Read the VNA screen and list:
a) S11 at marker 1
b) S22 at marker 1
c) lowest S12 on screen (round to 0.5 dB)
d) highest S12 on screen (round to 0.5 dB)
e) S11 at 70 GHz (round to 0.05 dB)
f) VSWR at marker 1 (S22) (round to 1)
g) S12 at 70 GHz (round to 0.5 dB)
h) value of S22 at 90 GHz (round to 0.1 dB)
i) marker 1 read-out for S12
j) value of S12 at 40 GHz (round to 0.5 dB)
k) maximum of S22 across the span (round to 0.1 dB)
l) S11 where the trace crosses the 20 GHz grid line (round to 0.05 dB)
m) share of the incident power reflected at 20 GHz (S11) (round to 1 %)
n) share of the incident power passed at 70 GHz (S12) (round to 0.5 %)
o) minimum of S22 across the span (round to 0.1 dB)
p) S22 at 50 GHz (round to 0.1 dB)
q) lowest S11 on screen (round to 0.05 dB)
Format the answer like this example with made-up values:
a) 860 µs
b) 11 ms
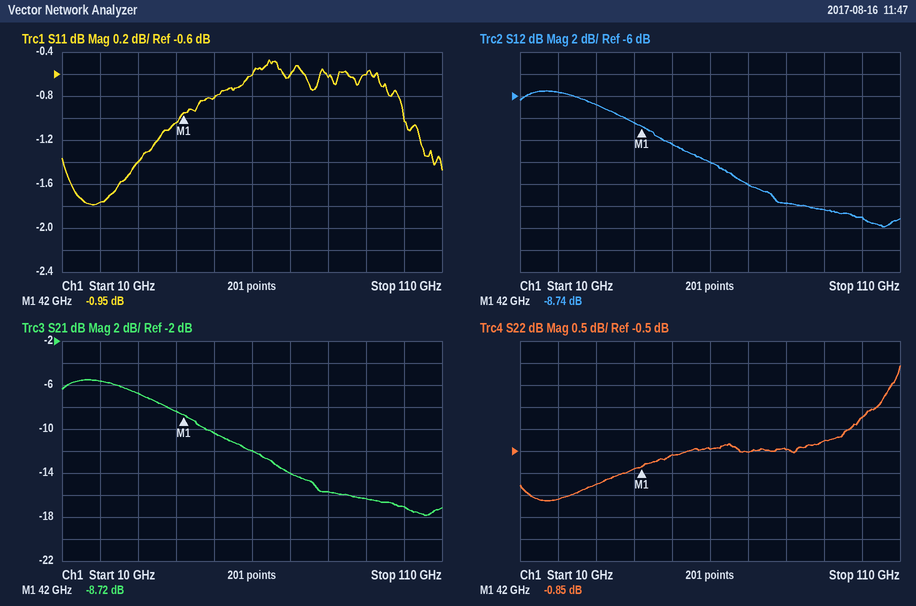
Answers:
a) -0.95 dB
b) -0.85 dB
c) -18.0 dB
d) -5.5 dB
e) -0.60 dB
f) 20
g) -14.0 dB
h) -0.3 dB
i) -8.74 dB
j) -8.5 dB
k) 1.4 dB
l) -1.75 dB
m) 67 %
n) 4.0 %
o) -1.6 dB
p) -0.6 dB
q) -1.80 dB
